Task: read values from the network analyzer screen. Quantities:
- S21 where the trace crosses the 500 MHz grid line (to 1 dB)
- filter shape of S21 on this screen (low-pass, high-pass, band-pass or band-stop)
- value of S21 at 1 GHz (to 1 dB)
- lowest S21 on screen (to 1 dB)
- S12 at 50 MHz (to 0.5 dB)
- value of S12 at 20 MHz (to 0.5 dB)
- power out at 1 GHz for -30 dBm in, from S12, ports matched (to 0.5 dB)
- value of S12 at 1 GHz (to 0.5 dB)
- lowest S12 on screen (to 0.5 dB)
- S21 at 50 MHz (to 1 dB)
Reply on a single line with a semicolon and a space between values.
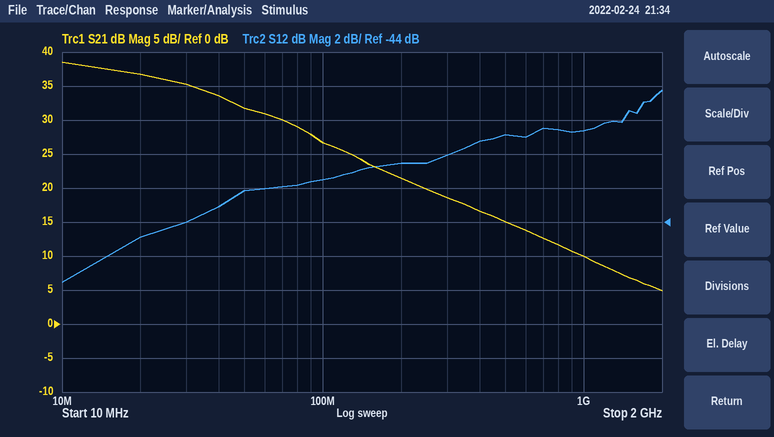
15 dB; low-pass; 10 dB; 5 dB; -42.0 dB; -45.0 dB; -68.5 dBm; -38.5 dB; -47.5 dB; 32 dB
